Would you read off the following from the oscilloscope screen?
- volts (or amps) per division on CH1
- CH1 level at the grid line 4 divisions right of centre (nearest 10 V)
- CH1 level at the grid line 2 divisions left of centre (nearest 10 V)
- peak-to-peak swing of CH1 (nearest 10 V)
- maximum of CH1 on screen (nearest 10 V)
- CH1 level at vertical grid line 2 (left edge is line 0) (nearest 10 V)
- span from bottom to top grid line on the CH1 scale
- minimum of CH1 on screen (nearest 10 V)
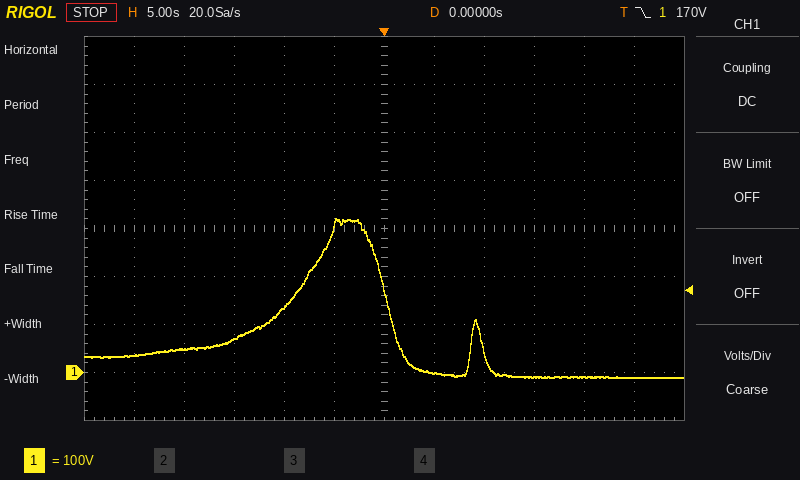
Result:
100 V
-10 V
140 V
330 V
320 V
50 V
800 V
-10 V
